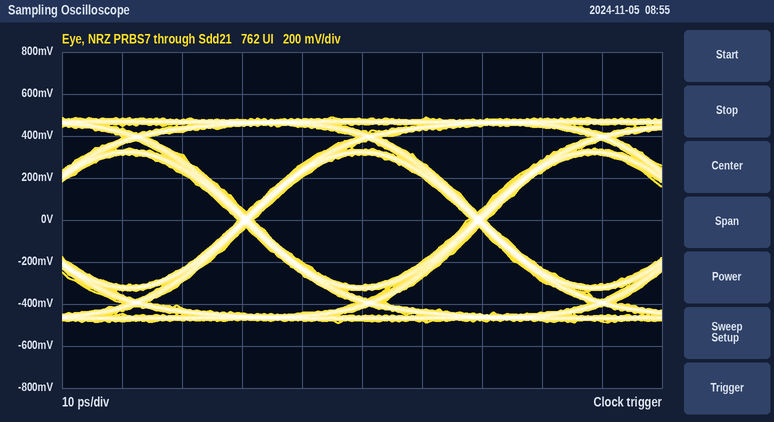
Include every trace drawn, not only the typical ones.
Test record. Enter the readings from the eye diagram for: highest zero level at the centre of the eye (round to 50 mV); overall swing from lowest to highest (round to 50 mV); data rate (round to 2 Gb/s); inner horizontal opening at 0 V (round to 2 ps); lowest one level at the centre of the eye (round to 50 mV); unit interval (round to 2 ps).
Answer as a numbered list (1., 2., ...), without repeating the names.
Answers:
1. -300 mV
2. 1.00 V
3. 26 Gb/s
4. 36 ps
5. 300 mV
6. 38 ps
